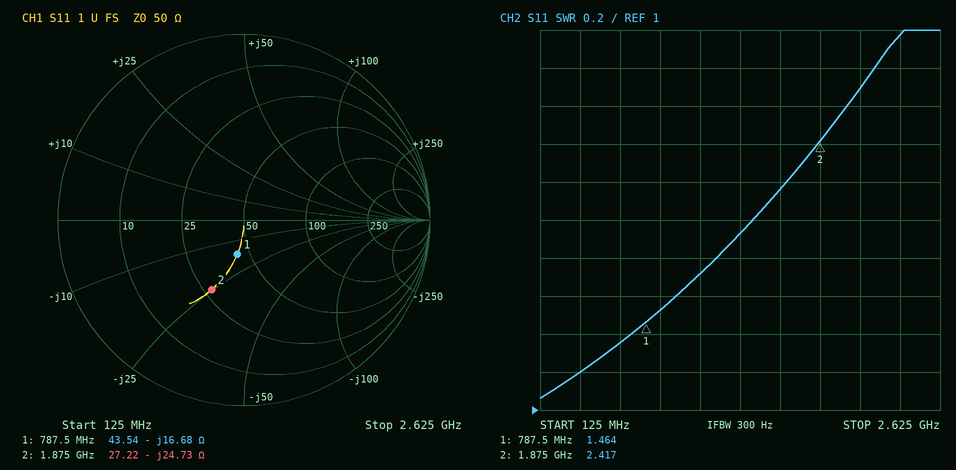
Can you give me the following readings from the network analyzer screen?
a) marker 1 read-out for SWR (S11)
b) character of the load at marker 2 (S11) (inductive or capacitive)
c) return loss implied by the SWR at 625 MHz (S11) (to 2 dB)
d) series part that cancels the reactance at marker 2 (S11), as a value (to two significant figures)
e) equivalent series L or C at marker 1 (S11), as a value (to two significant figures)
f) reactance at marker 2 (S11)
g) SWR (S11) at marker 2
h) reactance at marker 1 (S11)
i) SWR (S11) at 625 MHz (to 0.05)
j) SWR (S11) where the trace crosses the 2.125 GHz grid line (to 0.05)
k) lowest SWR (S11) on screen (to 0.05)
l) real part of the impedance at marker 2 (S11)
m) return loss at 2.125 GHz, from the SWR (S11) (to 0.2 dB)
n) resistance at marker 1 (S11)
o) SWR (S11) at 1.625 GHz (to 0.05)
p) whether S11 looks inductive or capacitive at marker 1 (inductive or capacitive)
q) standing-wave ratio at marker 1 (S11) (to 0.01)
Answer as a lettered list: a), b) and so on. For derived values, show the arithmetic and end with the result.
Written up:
a) 1.464
b) capacitive
c) −20 log10((1.35 − 1)/(1.35 + 1)) ≈ 16 dB
d) L = 24.73 Ω/(2π × 1.875 GHz) ≈ 2.1 nH
e) C = 1/(2π × 787.5 MHz × 16.68 Ω) ≈ 12 pF
f) -24.73 Ω
g) 2.417
h) -16.68 Ω
i) 1.35
j) 2.70
k) 1.05
l) 27.22 Ω
m) −20 log10((2.7 − 1)/(2.7 + 1)) ≈ 6.8 dB
n) 43.54 Ω
o) 2.15
p) capacitive
q) 1.46
